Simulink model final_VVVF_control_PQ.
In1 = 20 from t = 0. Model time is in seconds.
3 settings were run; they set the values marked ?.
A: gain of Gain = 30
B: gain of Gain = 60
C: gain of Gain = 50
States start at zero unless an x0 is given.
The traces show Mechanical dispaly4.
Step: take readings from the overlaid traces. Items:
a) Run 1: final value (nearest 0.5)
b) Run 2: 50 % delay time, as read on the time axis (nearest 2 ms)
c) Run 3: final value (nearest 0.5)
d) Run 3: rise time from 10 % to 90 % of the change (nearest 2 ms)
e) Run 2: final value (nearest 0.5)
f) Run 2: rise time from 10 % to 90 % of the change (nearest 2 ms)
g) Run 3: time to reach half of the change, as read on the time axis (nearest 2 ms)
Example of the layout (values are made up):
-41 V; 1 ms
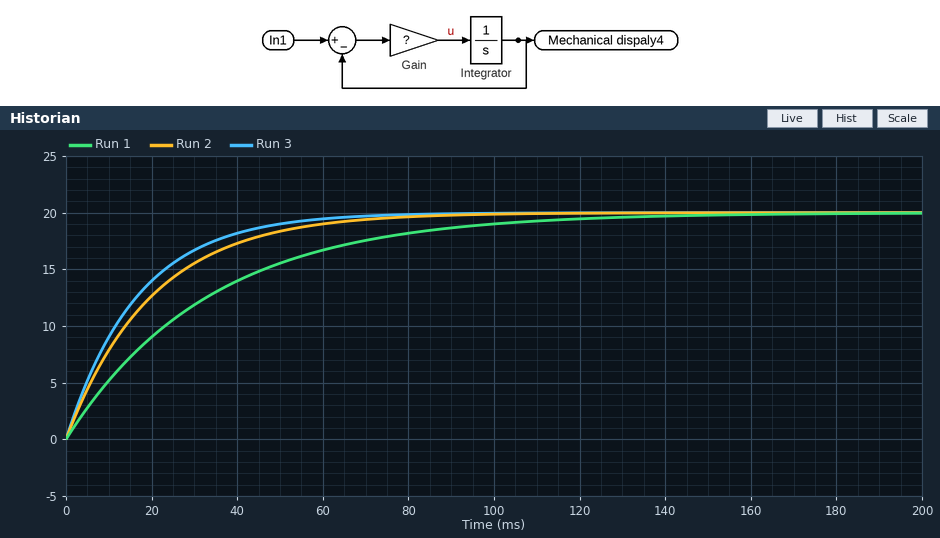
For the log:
20.0; 14 ms; 20.0; 36 ms; 20.0; 44 ms; 12 ms
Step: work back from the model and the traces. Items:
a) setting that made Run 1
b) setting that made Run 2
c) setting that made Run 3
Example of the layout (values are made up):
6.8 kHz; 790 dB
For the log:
A; C; B
